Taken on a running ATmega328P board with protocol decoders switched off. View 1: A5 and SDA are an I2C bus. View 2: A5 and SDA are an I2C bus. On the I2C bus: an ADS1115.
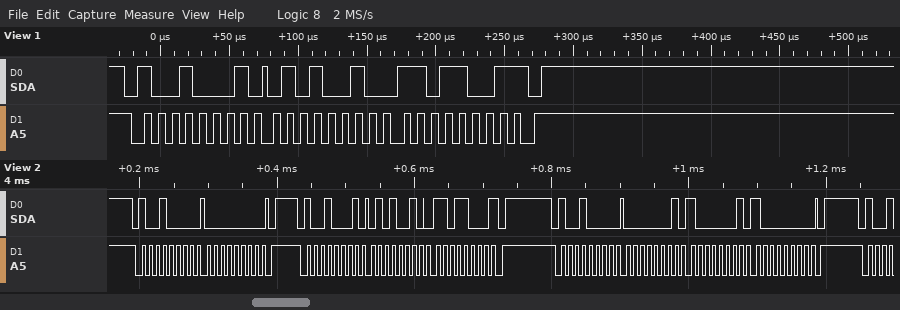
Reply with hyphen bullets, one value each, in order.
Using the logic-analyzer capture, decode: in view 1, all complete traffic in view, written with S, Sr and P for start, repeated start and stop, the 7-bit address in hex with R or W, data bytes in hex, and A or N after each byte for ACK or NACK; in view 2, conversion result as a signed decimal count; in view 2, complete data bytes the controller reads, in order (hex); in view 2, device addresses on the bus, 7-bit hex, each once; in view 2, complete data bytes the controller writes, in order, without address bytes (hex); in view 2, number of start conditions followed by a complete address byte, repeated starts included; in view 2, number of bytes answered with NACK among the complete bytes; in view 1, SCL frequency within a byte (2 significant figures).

- S 48R A 52 A D9 N P
- 21208
- 52 D8
- 0x48
- 00 01 81 80
- 3
- 1
- 100 kHz
